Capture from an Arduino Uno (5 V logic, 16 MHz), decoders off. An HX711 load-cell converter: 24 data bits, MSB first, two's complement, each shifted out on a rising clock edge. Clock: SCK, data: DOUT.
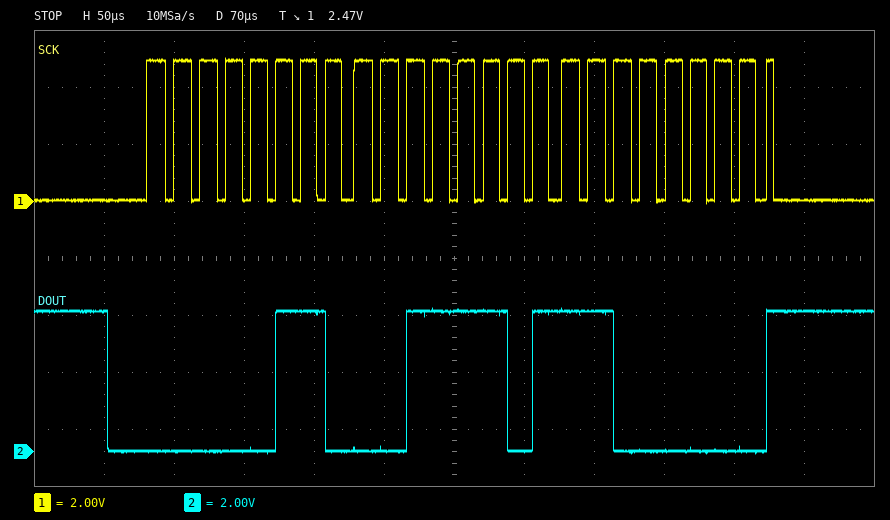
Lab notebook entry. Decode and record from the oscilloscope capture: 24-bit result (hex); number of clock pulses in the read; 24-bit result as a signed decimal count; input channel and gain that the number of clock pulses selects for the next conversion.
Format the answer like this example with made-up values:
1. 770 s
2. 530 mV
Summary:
1. 0x063DC0
2. 25
3. 409024
4. channel A, gain 128
